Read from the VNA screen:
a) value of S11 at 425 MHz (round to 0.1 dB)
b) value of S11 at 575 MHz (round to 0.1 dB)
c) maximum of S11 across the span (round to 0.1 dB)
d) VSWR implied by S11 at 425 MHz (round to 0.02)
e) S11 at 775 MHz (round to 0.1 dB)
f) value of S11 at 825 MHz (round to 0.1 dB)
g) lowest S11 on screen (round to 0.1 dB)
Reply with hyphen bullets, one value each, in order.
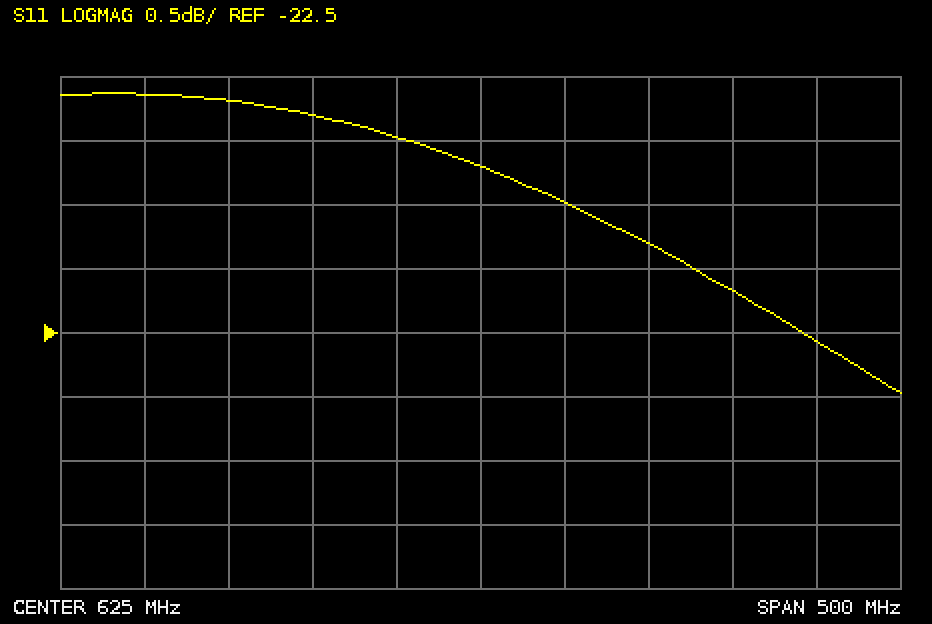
- -20.6 dB
- -21.0 dB
- -20.6 dB
- 1.20
- -22.2 dB
- -22.6 dB
- -23.0 dB
